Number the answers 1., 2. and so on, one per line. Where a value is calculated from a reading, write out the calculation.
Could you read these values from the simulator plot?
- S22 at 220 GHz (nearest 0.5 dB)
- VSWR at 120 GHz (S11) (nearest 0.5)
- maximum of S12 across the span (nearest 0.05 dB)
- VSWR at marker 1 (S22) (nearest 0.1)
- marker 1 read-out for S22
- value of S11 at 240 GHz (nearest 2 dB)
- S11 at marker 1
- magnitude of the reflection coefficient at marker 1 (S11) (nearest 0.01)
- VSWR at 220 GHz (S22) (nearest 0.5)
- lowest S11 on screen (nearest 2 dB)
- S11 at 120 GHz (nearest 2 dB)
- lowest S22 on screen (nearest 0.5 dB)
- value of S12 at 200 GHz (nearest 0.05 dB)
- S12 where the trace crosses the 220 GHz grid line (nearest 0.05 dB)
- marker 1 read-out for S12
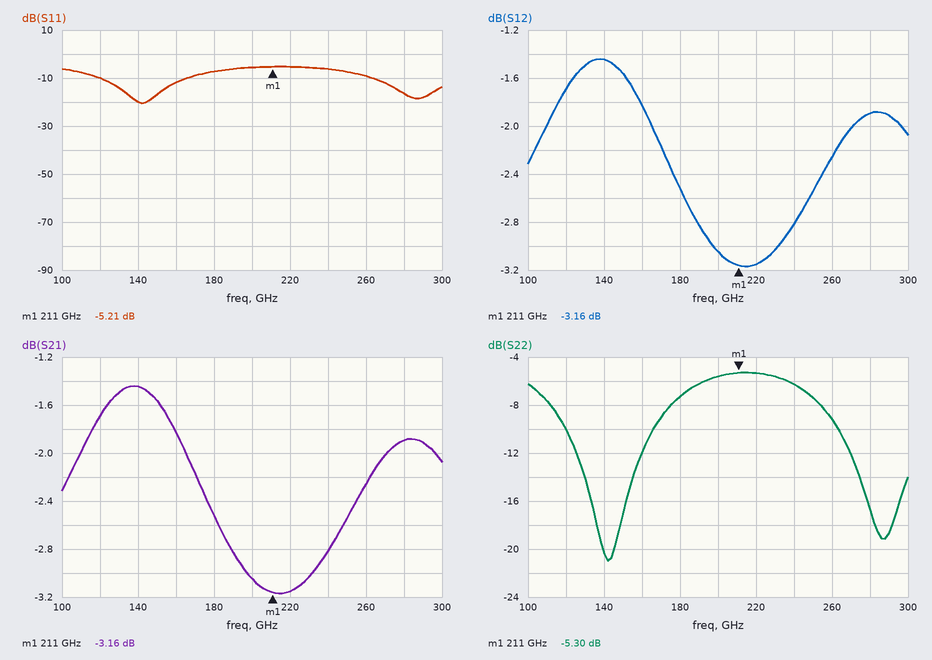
1. -5.5 dB
2. |Γ| = 10^(-10/20) = 0.3162; VSWR = (1 + 0.3162)/(1 − 0.3162) ≈ 1.92, so 2.0 to the nearest 0.5
3. -1.45 dB
4. (1 + 0.5433)/(1 − 0.5433) ≈ 3.4
5. -5.30 dB
6. -6 dB
7. -5.21 dB
8. 10^(-5.21/20) ≈ 0.55
9. |Γ| = 10^(-5.5/20) = 0.5309; VSWR = (1 + 0.5309)/(1 − 0.5309) ≈ 3.26, so 3.5 to the nearest 0.5
10. -20 dB
11. -10 dB
12. -21.0 dB
13. -3.05 dB
14. -3.15 dB
15. -3.16 dB
